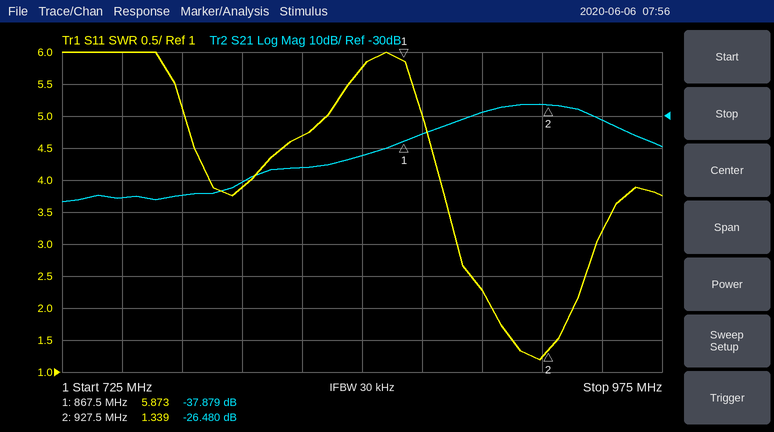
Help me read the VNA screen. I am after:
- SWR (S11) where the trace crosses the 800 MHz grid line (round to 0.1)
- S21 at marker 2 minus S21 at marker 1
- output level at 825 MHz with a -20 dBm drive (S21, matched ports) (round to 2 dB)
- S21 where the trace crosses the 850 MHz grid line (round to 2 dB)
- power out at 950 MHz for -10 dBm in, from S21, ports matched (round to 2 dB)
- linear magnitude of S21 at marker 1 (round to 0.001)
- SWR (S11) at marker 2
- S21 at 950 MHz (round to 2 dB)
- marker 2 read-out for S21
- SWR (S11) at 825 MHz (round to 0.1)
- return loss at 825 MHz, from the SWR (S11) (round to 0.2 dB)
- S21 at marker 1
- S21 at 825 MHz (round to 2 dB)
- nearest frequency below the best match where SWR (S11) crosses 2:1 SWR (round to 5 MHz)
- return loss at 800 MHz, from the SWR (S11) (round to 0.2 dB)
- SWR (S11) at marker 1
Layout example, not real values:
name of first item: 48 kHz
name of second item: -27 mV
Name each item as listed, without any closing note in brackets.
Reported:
SWR (S11) where the trace crosses the 800 MHz grid line: 3.9
S21 at marker 2 minus S21 at marker 1: 11.399 dB
output level at 825 MHz with a -20 dBm drive (S21, matched ports): -66 dBm
S21 where the trace crosses the 850 MHz grid line: -42 dB
power out at 950 MHz for -10 dBm in, from S21, ports matched: -42 dBm
linear magnitude of S21 at marker 1: 0.013
SWR (S11) at marker 2: 1.339
S21 at 950 MHz: -32 dB
marker 2 read-out for S21: -26.480 dB
SWR (S11) at 825 MHz: 4.7
return loss at 825 MHz, from the SWR (S11): 3.8 dB
S21 at marker 1: -37.879 dB
S21 at 825 MHz: -46 dB
nearest frequency below the best match where SWR (S11) crosses 2:1 SWR: 905 MHz
return loss at 800 MHz, from the SWR (S11): 4.6 dB
SWR (S11) at marker 1: 5.873
